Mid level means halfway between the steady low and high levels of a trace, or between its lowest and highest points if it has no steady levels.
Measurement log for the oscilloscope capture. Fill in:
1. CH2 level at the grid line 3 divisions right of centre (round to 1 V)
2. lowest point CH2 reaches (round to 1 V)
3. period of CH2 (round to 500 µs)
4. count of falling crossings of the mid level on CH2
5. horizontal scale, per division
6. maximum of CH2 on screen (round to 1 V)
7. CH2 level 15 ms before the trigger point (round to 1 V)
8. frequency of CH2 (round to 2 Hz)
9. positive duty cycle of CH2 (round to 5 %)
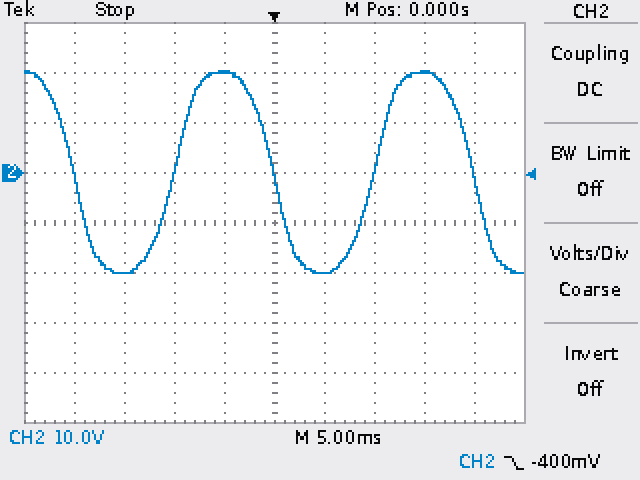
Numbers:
20 V
-20 V
20.0 ms
3
5 ms
20 V
-20 V
50 Hz
50 %
